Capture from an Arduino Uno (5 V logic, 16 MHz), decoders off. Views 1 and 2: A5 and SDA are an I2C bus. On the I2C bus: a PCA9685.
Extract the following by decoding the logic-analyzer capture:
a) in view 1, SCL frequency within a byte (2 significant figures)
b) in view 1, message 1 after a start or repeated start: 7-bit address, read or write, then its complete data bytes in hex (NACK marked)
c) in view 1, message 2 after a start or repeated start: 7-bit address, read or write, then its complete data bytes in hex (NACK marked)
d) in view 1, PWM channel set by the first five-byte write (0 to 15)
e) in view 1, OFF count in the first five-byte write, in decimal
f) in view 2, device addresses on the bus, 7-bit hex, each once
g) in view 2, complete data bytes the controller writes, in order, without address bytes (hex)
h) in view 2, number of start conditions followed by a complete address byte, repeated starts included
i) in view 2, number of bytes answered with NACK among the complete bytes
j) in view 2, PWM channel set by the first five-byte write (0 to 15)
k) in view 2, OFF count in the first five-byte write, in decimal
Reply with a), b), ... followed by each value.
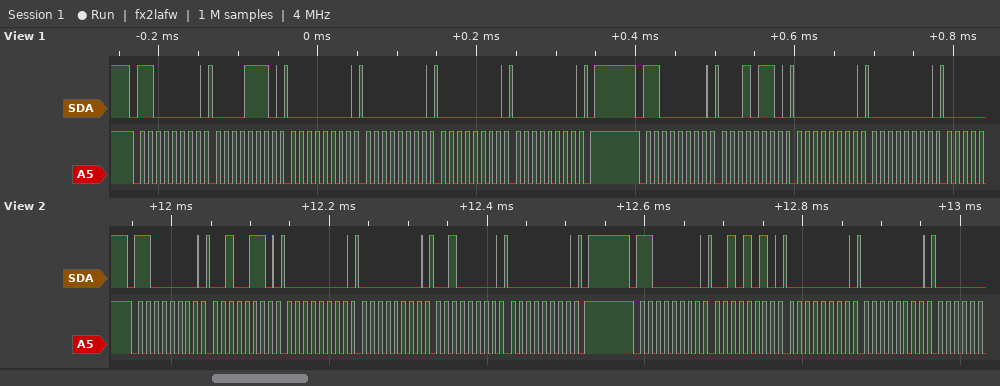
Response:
a) 100 kHz
b) 0x60 write: 0E 00 00 00 00
c) 0x60 write: 16 00 00
d) 2
e) 0
f) 0x60
g) 26 00 00 20 00 2A 00 00
h) 2
i) 0
j) 8
k) 32
